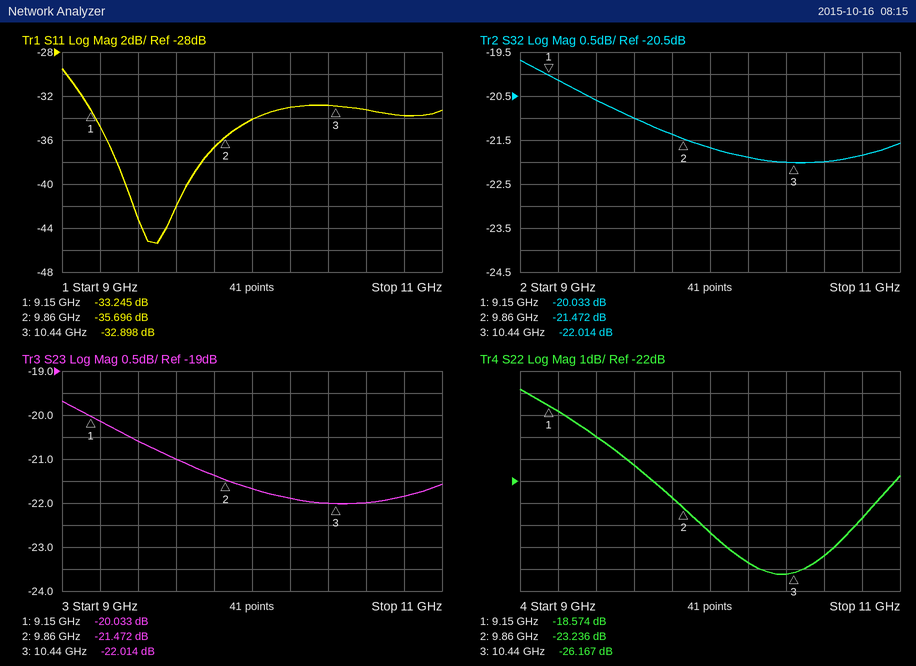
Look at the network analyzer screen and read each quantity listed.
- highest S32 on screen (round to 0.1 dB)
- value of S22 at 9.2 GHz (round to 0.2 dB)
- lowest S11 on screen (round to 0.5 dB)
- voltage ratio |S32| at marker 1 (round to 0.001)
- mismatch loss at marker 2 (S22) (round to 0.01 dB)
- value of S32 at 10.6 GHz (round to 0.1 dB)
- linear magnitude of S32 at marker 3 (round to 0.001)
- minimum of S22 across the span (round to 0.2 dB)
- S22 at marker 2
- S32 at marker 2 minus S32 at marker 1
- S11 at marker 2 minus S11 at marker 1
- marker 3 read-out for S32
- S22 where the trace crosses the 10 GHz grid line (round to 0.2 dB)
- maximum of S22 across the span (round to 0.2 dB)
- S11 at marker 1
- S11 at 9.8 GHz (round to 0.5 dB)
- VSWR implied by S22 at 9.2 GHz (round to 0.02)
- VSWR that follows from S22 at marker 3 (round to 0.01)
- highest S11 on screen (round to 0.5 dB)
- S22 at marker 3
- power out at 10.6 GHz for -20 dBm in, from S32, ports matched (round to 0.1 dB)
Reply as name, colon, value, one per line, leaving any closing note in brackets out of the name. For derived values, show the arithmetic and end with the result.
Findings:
highest S32 on screen: -19.7 dB
value of S22 at 9.2 GHz: -18.8 dB
lowest S11 on screen: -45.5 dB
voltage ratio |S32| at marker 1: 10^(-20.033/20) ≈ 0.100
mismatch loss at marker 2 (S22): −10 log10(1 − 10^(-23.236/10)) ≈ 0.02 dB
value of S32 at 10.6 GHz: -22.0 dB
linear magnitude of S32 at marker 3: 10^(-22.014/20) ≈ 0.079
minimum of S22 across the span: -26.2 dB
S22 at marker 2: -23.236 dB
S32 at marker 2 minus S32 at marker 1: -21.472 − (-20.033) = -1.439 dB
S11 at marker 2 minus S11 at marker 1: -35.696 − (-33.245) = -2.451 dB
marker 3 read-out for S32: -22.014 dB
S22 where the trace crosses the 10 GHz grid line: -24.4 dB
maximum of S22 across the span: -17.8 dB
S11 at marker 1: -33.245 dB
S11 at 9.8 GHz: -36.5 dB
VSWR implied by S22 at 9.2 GHz: |Γ| = 10^(-18.8/20) = 0.1148; VSWR = (1 + 0.1148)/(1 − 0.1148) ≈ 1.26
VSWR that follows from S22 at marker 3: (1 + 0.0492)/(1 − 0.0492) ≈ 1.10
highest S11 on screen: -29.5 dB
S22 at marker 3: -26.167 dB
power out at 10.6 GHz for -20 dBm in, from S32, ports matched: -20 dBm + (-22.0 dB) = -42.0 dBm
